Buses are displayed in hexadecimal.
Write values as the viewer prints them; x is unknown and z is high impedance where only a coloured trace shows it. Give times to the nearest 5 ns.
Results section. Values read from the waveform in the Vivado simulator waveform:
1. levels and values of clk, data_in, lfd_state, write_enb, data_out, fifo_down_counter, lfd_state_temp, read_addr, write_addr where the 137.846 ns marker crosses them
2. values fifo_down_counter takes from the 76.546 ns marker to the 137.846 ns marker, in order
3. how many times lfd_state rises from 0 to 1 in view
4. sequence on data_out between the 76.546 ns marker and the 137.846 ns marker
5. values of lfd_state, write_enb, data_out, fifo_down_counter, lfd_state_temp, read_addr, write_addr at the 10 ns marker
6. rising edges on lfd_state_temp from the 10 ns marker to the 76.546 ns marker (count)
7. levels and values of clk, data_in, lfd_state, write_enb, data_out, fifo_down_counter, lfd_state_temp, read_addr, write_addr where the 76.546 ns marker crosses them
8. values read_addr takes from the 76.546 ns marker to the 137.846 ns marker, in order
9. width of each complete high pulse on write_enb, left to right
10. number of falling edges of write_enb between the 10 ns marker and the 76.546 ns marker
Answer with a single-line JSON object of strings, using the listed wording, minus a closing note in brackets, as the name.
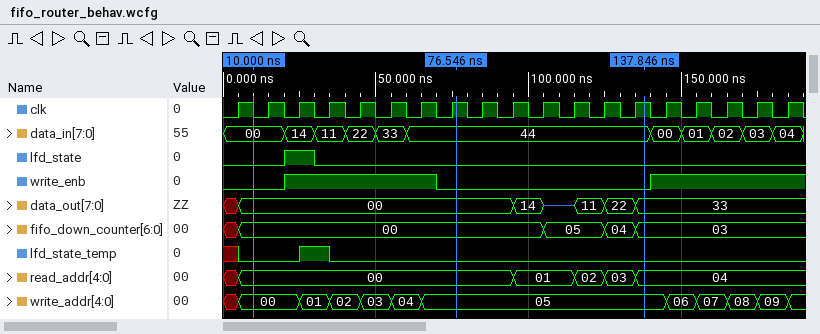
{"levels and values of clk, data_in, lfd_state, write_enb, data_out, fifo_down_counter, lfd_state_temp, read_addr, write_addr where the 137.846 ns marker crosses them": "clk=1, data_in=44, lfd_state=0, write_enb=0, data_out=33, fifo_down_counter=03, lfd_state_temp=0, read_addr=04, write_addr=05", "values fifo_down_counter takes from the 76.546 ns marker to the 137.846 ns marker, in order": "00, 05, 04, 03", "how many times lfd_state rises from 0 to 1 in view": "1", "sequence on data_out between the 76.546 ns marker and the 137.846 ns marker": "00, 14, z, 11, 22, 33", "values of lfd_state, write_enb, data_out, fifo_down_counter, lfd_state_temp, read_addr, write_addr at the 10 ns marker": "lfd_state=0, write_enb=0, data_out=00, fifo_down_counter=00, lfd_state_temp=0, read_addr=00, write_addr=00", "rising edges on lfd_state_temp from the 10 ns marker to the 76.546 ns marker": "1", "levels and values of clk, data_in, lfd_state, write_enb, data_out, fifo_down_counter, lfd_state_temp, read_addr, write_addr where the 76.546 ns marker crosses them": "clk=1, data_in=44, lfd_state=0, write_enb=0, data_out=00, fifo_down_counter=00, lfd_state_temp=0, read_addr=00, write_addr=05", "values read_addr takes from the 76.546 ns marker to the 137.846 ns marker, in order": "00, 01, 02, 03, 04", "width of each complete high pulse on write_enb, left to right": "50 ns", "number of falling edges of write_enb between the 10 ns marker and the 76.546 ns marker": "1"}
